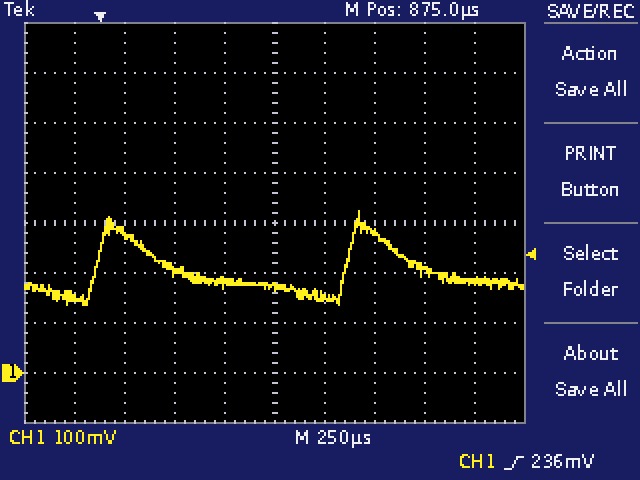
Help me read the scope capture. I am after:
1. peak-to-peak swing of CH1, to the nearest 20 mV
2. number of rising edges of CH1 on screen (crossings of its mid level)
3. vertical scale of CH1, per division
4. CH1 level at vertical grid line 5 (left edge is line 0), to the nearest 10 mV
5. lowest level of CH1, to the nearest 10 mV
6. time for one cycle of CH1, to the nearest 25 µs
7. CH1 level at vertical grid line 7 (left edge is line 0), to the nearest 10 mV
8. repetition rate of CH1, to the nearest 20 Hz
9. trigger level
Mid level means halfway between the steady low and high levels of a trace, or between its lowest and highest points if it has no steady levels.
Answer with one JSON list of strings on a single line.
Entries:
["180 mV", "2", "100 mV", "170 mV", "140 mV", "1.250 ms", "280 mV", "800 Hz", "236 mV"]
